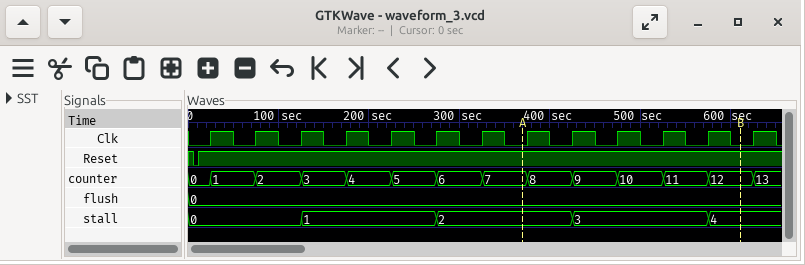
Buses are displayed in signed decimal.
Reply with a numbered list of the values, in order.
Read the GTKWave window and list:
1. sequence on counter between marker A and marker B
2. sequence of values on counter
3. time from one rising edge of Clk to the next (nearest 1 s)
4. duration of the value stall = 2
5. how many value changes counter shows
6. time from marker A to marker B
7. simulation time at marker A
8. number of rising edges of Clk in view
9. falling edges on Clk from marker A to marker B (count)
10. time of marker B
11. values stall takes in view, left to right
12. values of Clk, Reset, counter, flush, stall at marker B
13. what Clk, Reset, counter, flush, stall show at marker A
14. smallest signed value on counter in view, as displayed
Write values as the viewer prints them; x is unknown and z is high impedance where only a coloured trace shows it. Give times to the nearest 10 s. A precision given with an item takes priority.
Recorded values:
1. 7, 8, 9, 10, 11, 12
2. 0, 1, 2, 3, 4, 5, 6, 7, 8, 9, 10, 11, 12, 13
3. 50 s
4. 150 s
5. 13
6. 240 s
7. 370 s
8. 13
9. 5
10. 610 s
11. 0, 1, 2, 3, 4
12. Clk=0, Reset=1, counter=12, flush=0, stall=4
13. Clk=0, Reset=1, counter=7, flush=0, stall=2
14. 0
